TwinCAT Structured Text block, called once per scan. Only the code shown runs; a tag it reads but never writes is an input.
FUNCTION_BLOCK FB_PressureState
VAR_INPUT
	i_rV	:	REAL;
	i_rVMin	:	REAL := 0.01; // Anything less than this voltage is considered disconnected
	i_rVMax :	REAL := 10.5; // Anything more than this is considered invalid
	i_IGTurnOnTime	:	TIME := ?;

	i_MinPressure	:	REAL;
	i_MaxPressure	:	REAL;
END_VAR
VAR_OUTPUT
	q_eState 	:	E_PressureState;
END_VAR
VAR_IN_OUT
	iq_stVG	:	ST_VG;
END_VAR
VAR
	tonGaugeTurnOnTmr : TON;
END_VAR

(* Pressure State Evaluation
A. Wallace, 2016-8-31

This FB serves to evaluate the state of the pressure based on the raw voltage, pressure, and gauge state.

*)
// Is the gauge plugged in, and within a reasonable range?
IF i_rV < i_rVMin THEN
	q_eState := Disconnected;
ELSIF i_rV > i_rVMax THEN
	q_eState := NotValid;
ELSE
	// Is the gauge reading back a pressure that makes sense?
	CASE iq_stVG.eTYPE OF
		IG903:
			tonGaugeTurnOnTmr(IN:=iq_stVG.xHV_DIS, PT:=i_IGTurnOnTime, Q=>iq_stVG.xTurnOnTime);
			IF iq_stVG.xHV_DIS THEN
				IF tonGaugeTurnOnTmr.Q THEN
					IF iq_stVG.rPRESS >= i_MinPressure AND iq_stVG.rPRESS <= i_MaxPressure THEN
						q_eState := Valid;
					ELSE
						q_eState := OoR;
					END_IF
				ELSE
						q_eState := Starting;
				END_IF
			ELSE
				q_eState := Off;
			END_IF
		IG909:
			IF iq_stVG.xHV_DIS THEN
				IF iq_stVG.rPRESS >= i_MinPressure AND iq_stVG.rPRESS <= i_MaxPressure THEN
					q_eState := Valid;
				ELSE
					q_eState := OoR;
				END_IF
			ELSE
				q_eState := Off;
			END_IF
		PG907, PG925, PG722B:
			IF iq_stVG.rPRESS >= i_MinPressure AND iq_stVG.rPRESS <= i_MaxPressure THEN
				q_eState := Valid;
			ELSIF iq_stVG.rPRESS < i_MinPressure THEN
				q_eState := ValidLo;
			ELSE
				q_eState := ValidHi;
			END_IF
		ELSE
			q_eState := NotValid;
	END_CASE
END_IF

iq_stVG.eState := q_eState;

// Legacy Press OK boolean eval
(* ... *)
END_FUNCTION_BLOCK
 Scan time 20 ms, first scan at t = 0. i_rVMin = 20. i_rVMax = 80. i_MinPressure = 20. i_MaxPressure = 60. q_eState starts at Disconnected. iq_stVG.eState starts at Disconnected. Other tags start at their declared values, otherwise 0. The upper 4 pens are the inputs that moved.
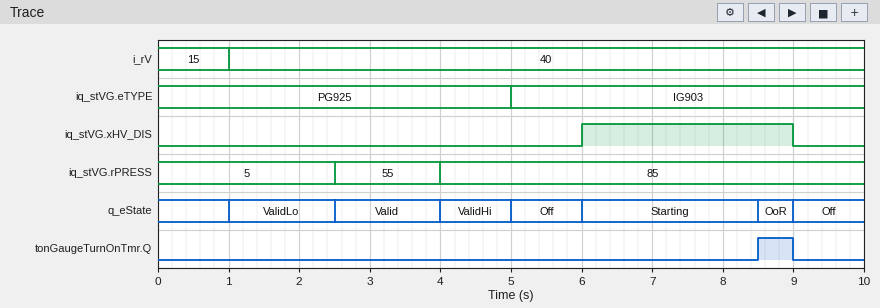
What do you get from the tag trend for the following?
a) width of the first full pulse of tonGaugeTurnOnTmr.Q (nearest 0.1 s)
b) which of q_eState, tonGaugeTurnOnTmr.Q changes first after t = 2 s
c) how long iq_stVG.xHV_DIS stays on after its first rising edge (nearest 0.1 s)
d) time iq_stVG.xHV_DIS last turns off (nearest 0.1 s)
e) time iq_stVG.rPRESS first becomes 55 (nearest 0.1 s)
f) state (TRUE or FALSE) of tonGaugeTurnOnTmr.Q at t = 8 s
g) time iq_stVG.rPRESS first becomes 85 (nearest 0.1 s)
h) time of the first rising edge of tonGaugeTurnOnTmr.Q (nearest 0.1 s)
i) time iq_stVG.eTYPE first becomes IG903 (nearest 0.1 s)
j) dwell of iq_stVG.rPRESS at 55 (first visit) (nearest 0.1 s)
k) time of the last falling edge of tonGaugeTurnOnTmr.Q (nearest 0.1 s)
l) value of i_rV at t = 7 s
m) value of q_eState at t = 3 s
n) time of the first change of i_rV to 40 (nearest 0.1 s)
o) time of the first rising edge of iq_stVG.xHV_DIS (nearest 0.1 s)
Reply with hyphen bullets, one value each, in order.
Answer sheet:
- 0.5 s
- q_eState
- 3.0 s
- 9.0 s
- 2.5 s
- FALSE
- 4.0 s
- 8.5 s
- 5.0 s
- 1.5 s
- 9.0 s
- 40
- Valid
- 1.0 s
- 6.0 s
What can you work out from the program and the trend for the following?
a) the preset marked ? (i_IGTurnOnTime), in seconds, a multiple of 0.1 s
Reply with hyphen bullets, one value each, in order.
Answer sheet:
- 2.5 s
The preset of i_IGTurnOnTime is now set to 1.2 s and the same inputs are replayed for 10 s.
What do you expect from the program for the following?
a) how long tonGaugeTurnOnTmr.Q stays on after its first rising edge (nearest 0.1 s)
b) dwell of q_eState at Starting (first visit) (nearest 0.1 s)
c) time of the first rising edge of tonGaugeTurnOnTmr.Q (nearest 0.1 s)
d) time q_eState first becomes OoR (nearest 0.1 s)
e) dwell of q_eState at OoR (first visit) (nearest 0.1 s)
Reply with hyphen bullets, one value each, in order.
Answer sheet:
- 1.8 s
- 1.2 s
- 7.2 s
- 7.2 s
- 1.8 s
